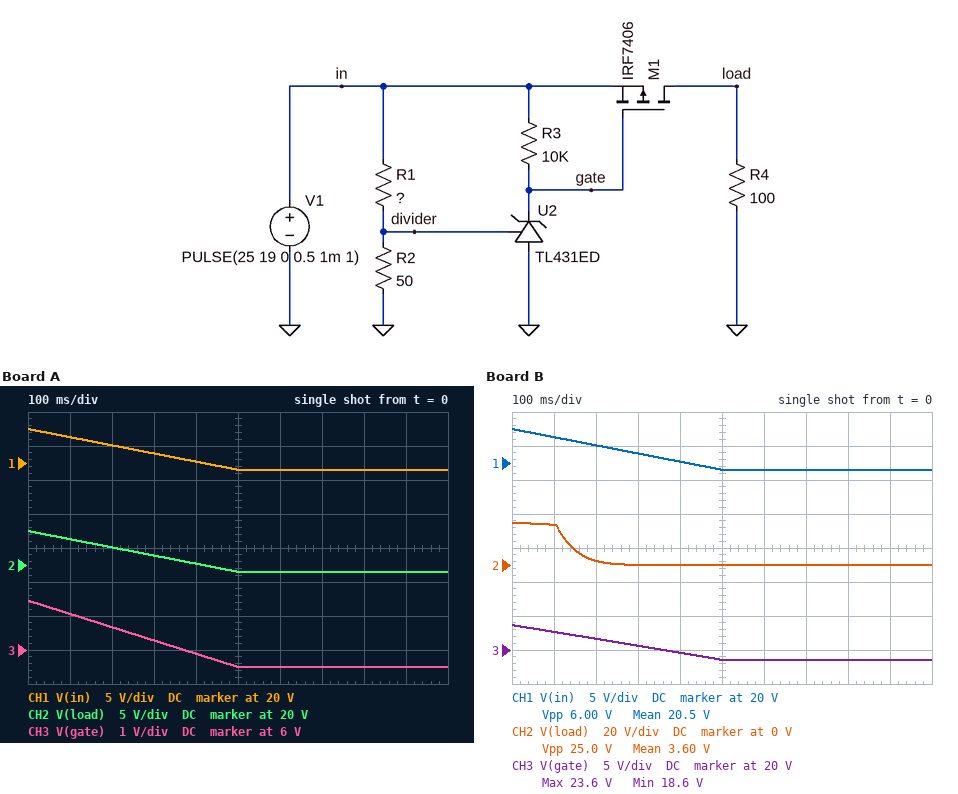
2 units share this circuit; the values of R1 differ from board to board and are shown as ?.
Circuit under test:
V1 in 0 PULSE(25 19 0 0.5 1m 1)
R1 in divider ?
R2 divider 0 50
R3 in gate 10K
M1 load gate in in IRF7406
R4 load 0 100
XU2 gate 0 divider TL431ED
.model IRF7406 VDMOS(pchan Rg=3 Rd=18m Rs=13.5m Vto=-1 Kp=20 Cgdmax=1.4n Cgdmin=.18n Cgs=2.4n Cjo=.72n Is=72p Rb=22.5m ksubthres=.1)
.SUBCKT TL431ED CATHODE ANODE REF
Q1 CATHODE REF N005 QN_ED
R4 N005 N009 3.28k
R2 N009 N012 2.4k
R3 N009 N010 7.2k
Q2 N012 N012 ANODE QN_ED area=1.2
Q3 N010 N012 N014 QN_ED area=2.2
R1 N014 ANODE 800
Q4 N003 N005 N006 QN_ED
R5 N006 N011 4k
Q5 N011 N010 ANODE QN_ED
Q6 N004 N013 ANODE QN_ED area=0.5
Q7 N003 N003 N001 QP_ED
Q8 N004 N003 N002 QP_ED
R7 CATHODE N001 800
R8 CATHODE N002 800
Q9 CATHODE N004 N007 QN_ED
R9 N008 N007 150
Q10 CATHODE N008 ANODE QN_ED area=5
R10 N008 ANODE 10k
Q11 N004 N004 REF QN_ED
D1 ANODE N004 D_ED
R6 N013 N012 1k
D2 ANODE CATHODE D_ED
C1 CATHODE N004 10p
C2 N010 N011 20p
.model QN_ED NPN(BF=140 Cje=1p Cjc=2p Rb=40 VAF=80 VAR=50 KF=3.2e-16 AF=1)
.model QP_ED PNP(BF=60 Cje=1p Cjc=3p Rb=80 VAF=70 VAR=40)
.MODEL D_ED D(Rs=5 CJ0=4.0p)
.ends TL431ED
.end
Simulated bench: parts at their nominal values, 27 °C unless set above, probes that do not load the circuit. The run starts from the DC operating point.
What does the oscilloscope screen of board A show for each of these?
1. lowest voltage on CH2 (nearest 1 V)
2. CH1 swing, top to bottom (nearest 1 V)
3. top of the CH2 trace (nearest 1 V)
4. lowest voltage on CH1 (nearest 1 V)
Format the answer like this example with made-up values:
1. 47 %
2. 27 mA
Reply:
1. 19 V
2. 6 V
3. 25 V
4. 19 V
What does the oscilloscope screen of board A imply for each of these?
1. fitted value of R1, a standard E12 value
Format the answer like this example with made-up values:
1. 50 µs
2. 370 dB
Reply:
1. 100 Ω
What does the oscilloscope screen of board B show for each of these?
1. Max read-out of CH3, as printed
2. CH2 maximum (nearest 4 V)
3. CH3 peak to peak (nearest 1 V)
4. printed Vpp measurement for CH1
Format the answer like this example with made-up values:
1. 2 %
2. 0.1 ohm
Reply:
1. 23.6 V
2. 24 V
3. 5 V
4. 6.00 V
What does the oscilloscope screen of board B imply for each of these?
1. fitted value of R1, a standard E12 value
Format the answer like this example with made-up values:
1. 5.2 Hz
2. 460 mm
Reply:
1. 560 Ω
